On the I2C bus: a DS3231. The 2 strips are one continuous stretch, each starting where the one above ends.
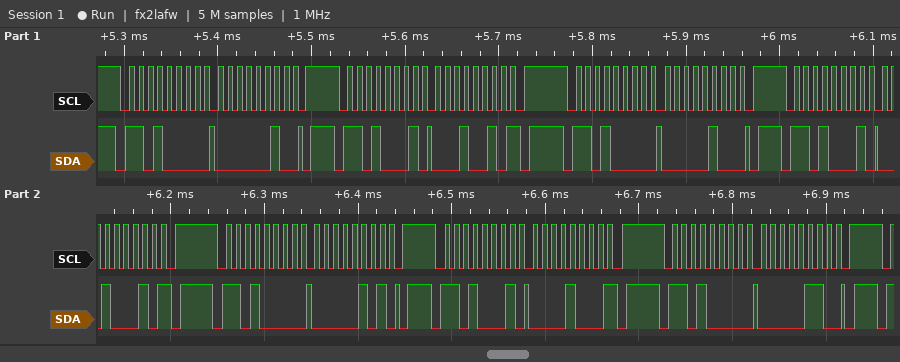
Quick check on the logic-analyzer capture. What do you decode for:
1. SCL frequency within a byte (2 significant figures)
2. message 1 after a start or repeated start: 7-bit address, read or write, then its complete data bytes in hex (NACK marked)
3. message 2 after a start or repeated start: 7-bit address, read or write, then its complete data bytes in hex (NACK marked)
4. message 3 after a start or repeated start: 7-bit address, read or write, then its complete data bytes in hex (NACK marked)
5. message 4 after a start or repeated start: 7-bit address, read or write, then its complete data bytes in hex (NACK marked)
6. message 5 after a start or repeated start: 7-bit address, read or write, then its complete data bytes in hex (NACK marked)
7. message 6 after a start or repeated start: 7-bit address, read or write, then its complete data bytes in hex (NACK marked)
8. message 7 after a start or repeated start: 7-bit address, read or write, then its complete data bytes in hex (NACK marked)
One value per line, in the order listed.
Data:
100 kHz
0x68 write: 02
0x68 read: 12 NACK
0x68 write: 04
0x68 read: 22 NACK
0x68 write: 05
0x68 read: 08 NACK
0x68 write: 06
